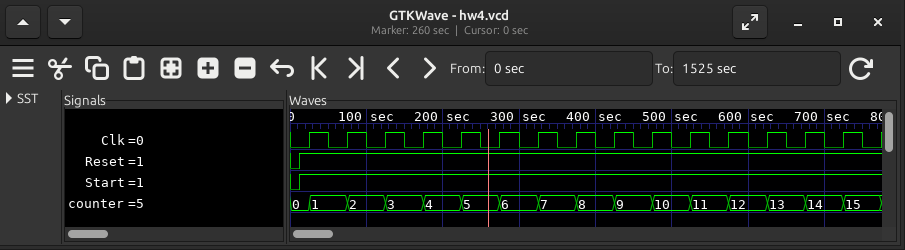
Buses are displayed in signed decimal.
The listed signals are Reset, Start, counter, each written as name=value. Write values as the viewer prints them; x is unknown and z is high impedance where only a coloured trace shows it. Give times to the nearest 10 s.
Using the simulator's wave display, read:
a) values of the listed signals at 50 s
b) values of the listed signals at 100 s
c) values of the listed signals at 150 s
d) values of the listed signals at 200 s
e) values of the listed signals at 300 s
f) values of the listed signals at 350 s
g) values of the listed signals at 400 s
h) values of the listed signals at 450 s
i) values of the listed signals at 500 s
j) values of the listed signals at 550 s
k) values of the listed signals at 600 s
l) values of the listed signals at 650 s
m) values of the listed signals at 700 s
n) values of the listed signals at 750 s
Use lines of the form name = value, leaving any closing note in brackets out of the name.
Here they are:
values of the listed signals at 50 s = Reset=1, Start=1, counter=1
values of the listed signals at 100 s = Reset=1, Start=1, counter=2
values of the listed signals at 150 s = Reset=1, Start=1, counter=3
values of the listed signals at 200 s = Reset=1, Start=1, counter=4
values of the listed signals at 300 s = Reset=1, Start=1, counter=6
values of the listed signals at 350 s = Reset=1, Start=1, counter=7
values of the listed signals at 400 s = Reset=1, Start=1, counter=8
values of the listed signals at 450 s = Reset=1, Start=1, counter=9
values of the listed signals at 500 s = Reset=1, Start=1, counter=10
values of the listed signals at 550 s = Reset=1, Start=1, counter=11
values of the listed signals at 600 s = Reset=1, Start=1, counter=12
values of the listed signals at 650 s = Reset=1, Start=1, counter=13
values of the listed signals at 700 s = Reset=1, Start=1, counter=14
values of the listed signals at 750 s = Reset=1, Start=1, counter=15
